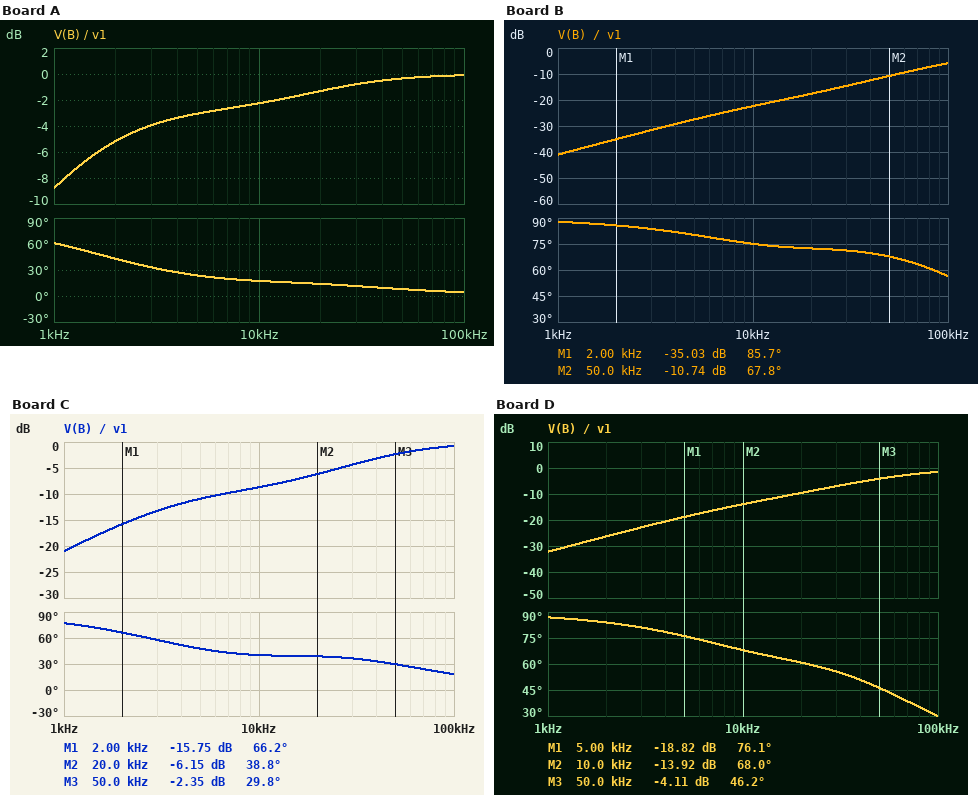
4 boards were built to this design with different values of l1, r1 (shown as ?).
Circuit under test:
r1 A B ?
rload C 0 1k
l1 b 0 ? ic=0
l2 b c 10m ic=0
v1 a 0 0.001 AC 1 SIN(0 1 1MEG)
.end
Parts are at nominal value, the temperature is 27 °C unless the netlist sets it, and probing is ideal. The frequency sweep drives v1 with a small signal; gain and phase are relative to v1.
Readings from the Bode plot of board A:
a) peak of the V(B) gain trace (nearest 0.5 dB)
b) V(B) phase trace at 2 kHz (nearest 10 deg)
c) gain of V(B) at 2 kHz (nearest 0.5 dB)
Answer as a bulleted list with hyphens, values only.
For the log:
- 0 dB
- 40 deg
- -5.0 dB
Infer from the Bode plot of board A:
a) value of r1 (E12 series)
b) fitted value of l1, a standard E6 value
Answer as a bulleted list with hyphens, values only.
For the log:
- 330 Ω
- 22 mH
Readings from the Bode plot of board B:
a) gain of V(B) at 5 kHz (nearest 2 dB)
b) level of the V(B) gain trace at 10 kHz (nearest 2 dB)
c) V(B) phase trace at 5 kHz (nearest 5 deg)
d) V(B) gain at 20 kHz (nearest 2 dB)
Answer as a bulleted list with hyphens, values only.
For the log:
- -28 dB
- -22 dB
- 80 deg
- -18 dB
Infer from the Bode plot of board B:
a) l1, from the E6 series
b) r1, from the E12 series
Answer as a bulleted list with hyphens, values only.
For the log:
- 4.7 mH
- 3.3 kΩ
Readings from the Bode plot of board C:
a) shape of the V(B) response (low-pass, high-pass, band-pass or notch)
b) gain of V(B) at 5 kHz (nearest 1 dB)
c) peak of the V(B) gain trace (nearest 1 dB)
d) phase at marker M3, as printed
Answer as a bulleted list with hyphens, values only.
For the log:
- high-pass
- -11 dB
- -1 dB
- 29.8 deg
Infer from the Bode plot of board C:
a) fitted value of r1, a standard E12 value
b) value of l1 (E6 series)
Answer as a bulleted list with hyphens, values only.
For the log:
- 1.5 kΩ
- 22 mH
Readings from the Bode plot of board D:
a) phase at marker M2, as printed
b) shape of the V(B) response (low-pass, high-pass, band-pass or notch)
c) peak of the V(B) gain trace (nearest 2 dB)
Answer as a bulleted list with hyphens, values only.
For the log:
- 68.0 deg
- high-pass
- -2 dB
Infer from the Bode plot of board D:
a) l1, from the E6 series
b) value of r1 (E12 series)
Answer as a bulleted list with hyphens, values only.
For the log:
- 4.7 mH
- 1.2 kΩ
